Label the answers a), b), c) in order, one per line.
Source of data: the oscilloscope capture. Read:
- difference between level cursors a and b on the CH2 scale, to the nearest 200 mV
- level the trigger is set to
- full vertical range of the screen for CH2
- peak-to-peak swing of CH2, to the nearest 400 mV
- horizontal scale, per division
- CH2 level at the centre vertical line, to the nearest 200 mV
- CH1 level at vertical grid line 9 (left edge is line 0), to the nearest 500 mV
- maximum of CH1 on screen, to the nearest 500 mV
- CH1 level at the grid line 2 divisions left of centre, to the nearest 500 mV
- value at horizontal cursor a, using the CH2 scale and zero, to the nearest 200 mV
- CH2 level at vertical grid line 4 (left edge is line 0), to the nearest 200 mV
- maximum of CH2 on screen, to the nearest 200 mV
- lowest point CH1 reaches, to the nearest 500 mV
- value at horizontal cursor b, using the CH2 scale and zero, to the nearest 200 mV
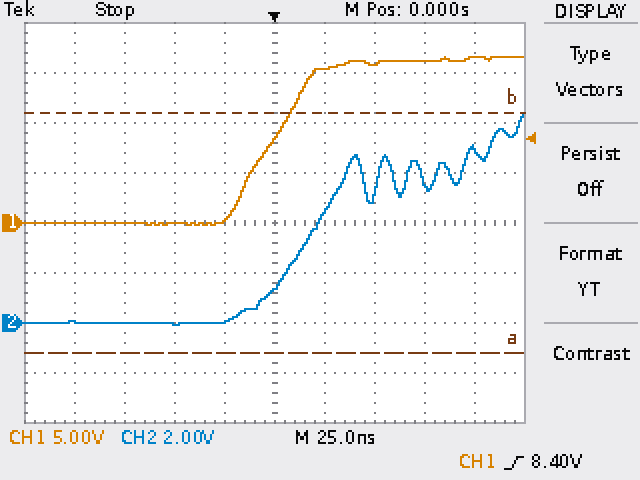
a) 9.6 V
b) 8.40 V
c) 16 V
d) 8.4 V
e) 25 ns
f) 1.4 V
g) 16.5 V
h) 16.5 V
i) 0.0 V
j) -1.2 V
k) 0.0 V
l) 8.4 V
m) 0.0 V
n) 8.4 V
